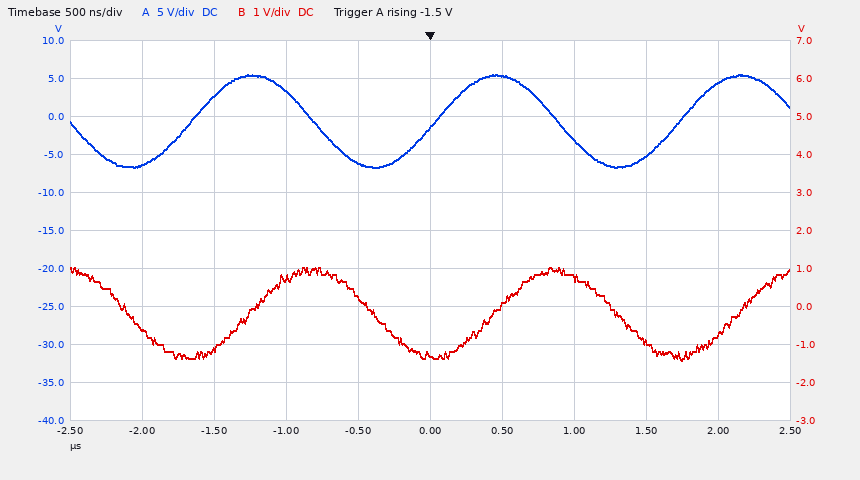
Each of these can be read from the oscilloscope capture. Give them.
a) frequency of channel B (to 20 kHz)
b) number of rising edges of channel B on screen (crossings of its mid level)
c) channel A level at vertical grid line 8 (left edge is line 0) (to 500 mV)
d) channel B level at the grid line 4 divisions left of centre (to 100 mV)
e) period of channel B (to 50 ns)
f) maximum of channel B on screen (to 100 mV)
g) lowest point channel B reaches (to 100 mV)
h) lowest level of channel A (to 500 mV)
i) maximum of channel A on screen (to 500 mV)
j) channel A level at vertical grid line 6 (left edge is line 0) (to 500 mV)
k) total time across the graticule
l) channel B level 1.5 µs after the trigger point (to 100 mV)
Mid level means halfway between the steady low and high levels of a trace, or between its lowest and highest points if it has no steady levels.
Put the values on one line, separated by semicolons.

580 kHz; 3; -5.0 V; -600 mV; 1.70 µs; 1.0 V; -1.4 V; -6.5 V; 5.5 V; 5.5 V; 5 µs; -900 mV
